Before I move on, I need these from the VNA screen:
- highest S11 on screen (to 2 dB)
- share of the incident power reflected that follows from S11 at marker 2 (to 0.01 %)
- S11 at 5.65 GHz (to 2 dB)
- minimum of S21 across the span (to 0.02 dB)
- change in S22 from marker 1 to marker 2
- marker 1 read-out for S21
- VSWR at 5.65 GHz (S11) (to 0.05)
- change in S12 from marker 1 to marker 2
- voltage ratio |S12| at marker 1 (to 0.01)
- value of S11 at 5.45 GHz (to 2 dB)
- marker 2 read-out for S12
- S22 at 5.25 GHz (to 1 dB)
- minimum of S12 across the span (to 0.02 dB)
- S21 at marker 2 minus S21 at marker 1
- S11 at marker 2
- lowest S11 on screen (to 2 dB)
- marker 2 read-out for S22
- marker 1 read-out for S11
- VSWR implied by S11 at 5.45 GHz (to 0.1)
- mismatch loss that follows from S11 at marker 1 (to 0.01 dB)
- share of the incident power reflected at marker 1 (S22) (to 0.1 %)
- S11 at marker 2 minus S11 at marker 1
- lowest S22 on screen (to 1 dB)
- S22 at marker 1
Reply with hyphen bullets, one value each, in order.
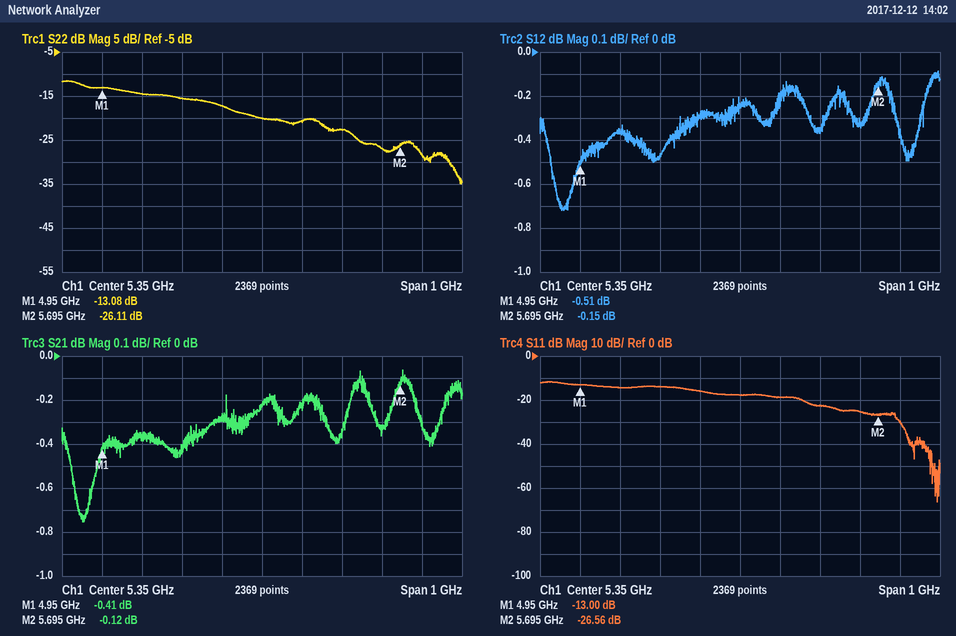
- -12 dB
- 0.22 %
- -26 dB
- -0.76 dB
- -13.03 dB
- -0.41 dB
- 1.10
- 0.36 dB
- 0.94
- -18 dB
- -0.15 dB
- -17 dB
- -0.72 dB
- 0.29 dB
- -26.56 dB
- -66 dB
- -26.11 dB
- -13.00 dB
- 1.3
- 0.22 dB
- 4.9 %
- -13.56 dB
- -35 dB
- -13.08 dB
